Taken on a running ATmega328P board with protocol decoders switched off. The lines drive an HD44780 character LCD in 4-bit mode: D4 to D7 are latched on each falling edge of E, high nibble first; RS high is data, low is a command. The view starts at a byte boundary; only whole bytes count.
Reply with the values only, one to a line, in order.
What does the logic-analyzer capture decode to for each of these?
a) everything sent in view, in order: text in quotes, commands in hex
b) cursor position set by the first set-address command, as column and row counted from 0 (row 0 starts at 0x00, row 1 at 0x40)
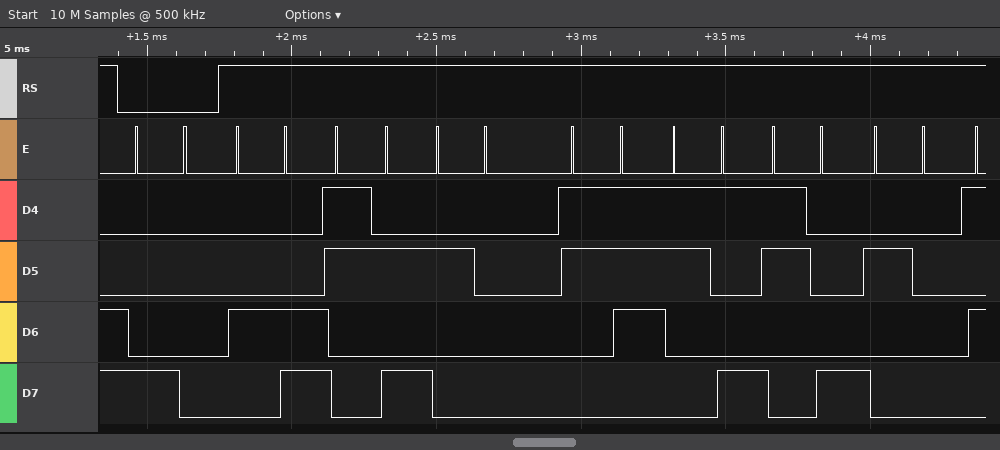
0x80 "L: 798 "
column 0, row 0
